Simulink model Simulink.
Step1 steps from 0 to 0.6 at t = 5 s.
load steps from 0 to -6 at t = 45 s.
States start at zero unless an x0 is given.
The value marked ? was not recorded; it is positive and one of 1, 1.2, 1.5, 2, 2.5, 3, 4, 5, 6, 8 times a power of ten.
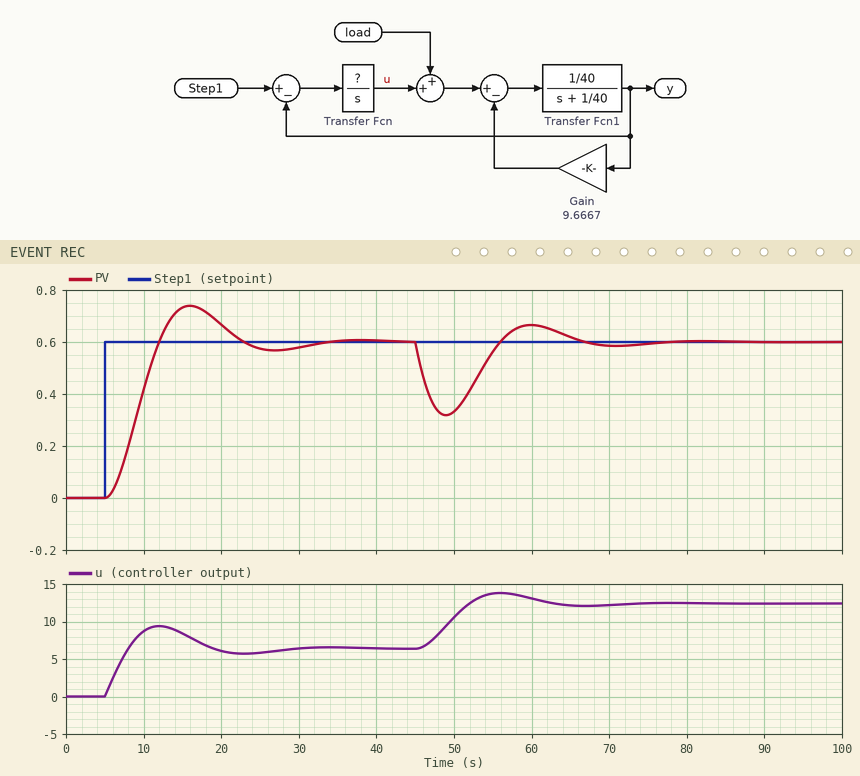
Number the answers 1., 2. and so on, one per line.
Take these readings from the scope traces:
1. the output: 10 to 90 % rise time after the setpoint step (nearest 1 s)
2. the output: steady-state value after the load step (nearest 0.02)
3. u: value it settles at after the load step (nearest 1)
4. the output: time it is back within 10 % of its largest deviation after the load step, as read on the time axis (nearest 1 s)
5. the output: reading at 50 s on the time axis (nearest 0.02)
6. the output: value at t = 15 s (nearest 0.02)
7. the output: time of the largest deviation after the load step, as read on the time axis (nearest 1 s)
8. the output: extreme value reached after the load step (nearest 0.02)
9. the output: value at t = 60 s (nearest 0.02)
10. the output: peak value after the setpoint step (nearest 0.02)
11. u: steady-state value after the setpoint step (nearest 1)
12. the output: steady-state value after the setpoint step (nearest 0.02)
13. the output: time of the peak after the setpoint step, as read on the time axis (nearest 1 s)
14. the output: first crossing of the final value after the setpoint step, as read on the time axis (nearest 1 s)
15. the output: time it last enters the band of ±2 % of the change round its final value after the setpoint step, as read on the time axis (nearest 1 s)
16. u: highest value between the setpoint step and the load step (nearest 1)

1. 5 s
2. 0.60
3. 12
4. 64 s
5. 0.34
6. 0.74
7. 49 s
8. 0.32
9. 0.66
10. 0.74
11. 6
12. 0.60
13. 16 s
14. 12 s
15. 32 s
16. 9
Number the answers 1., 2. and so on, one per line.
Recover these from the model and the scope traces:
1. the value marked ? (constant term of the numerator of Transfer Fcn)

1. 4
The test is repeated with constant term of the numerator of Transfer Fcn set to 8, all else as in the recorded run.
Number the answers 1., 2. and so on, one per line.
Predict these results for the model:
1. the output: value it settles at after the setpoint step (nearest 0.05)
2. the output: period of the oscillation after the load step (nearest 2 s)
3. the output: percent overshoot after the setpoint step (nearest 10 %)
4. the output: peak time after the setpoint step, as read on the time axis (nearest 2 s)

1. 0.60
2. 14 s
3. 40 %
4. 12 s
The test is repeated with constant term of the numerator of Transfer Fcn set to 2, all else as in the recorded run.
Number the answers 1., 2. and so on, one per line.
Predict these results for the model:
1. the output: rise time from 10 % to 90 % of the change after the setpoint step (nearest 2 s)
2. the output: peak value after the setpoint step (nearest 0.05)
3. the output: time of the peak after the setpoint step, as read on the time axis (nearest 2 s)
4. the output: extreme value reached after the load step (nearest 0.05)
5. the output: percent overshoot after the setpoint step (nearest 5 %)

1. 8 s
2. 0.65
3. 22 s
4. 0.25
5. 10 %
